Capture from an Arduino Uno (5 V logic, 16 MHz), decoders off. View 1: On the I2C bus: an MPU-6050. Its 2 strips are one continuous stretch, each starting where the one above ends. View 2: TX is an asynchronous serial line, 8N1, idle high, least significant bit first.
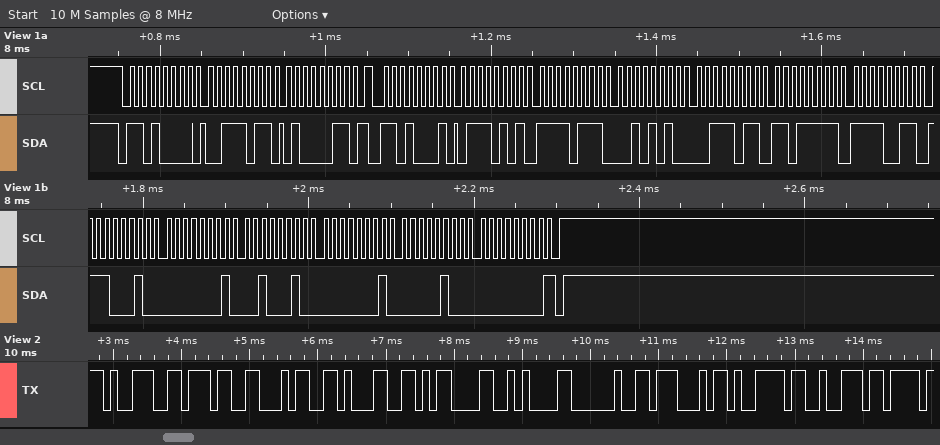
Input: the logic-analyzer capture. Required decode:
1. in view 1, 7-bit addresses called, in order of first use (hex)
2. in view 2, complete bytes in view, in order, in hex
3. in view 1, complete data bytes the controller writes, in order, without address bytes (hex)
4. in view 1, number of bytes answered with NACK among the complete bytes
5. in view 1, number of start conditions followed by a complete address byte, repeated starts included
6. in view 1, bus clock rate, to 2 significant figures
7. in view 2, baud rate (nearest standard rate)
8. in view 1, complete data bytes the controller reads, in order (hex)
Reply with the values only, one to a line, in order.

0x68
39 37 34 31 0D 0A 20 47 79 72
3B 43
1
2
100 kHz
9600 baud
75 F7 2A 3B DF F3 E2 01 22 01 04 00
